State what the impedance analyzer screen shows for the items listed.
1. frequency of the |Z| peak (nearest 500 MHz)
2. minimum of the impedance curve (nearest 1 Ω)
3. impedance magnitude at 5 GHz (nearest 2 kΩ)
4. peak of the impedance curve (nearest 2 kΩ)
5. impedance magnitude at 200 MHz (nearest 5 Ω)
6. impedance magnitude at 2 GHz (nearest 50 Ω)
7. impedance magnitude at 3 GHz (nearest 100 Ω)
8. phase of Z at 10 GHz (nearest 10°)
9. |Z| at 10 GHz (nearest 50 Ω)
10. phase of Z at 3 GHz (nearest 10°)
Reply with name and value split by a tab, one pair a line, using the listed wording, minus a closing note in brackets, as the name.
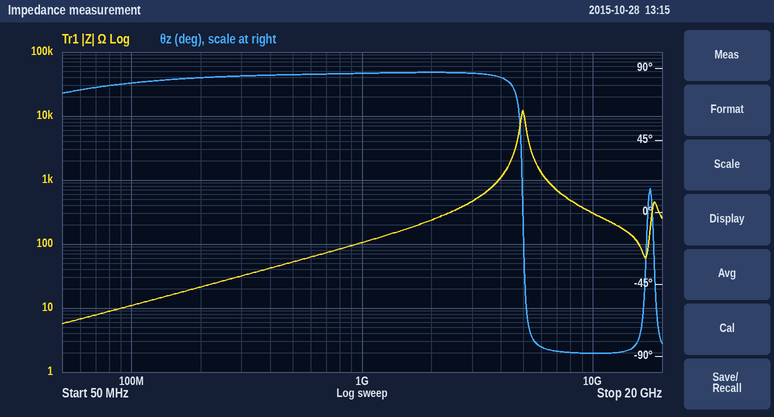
frequency of the |Z| peak	5.0 GHz
minimum of the impedance curve	6 Ω
impedance magnitude at 5 GHz	12 kΩ
peak of the impedance curve	12 kΩ
impedance magnitude at 200 MHz	20 Ω
impedance magnitude at 2 GHz	250 Ω
impedance magnitude at 3 GHz	500 Ω
phase of Z at 10 GHz	-90°
|Z| at 10 GHz	300 Ω
phase of Z at 3 GHz	90°
